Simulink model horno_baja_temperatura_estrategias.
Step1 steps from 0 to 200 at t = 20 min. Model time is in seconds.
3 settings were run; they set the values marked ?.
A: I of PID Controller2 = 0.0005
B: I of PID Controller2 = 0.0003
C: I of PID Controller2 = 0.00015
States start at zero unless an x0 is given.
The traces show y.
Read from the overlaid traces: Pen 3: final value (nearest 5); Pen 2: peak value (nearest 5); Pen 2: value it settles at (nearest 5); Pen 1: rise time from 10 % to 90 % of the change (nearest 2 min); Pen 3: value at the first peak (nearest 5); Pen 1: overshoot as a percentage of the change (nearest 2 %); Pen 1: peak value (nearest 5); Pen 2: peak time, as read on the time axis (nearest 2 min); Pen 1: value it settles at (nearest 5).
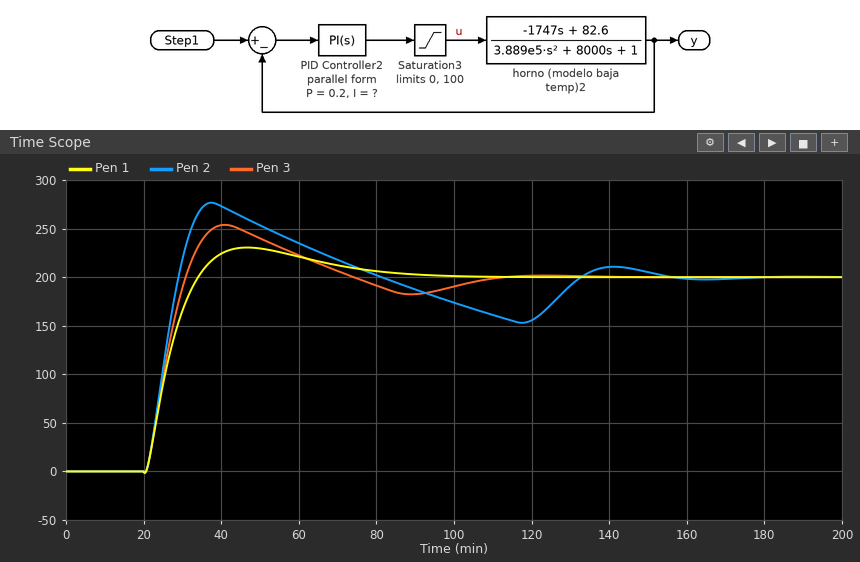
200
275
200
10 min
255
16 %
230
38 min
200
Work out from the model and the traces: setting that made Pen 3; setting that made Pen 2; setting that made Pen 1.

B
A
C
